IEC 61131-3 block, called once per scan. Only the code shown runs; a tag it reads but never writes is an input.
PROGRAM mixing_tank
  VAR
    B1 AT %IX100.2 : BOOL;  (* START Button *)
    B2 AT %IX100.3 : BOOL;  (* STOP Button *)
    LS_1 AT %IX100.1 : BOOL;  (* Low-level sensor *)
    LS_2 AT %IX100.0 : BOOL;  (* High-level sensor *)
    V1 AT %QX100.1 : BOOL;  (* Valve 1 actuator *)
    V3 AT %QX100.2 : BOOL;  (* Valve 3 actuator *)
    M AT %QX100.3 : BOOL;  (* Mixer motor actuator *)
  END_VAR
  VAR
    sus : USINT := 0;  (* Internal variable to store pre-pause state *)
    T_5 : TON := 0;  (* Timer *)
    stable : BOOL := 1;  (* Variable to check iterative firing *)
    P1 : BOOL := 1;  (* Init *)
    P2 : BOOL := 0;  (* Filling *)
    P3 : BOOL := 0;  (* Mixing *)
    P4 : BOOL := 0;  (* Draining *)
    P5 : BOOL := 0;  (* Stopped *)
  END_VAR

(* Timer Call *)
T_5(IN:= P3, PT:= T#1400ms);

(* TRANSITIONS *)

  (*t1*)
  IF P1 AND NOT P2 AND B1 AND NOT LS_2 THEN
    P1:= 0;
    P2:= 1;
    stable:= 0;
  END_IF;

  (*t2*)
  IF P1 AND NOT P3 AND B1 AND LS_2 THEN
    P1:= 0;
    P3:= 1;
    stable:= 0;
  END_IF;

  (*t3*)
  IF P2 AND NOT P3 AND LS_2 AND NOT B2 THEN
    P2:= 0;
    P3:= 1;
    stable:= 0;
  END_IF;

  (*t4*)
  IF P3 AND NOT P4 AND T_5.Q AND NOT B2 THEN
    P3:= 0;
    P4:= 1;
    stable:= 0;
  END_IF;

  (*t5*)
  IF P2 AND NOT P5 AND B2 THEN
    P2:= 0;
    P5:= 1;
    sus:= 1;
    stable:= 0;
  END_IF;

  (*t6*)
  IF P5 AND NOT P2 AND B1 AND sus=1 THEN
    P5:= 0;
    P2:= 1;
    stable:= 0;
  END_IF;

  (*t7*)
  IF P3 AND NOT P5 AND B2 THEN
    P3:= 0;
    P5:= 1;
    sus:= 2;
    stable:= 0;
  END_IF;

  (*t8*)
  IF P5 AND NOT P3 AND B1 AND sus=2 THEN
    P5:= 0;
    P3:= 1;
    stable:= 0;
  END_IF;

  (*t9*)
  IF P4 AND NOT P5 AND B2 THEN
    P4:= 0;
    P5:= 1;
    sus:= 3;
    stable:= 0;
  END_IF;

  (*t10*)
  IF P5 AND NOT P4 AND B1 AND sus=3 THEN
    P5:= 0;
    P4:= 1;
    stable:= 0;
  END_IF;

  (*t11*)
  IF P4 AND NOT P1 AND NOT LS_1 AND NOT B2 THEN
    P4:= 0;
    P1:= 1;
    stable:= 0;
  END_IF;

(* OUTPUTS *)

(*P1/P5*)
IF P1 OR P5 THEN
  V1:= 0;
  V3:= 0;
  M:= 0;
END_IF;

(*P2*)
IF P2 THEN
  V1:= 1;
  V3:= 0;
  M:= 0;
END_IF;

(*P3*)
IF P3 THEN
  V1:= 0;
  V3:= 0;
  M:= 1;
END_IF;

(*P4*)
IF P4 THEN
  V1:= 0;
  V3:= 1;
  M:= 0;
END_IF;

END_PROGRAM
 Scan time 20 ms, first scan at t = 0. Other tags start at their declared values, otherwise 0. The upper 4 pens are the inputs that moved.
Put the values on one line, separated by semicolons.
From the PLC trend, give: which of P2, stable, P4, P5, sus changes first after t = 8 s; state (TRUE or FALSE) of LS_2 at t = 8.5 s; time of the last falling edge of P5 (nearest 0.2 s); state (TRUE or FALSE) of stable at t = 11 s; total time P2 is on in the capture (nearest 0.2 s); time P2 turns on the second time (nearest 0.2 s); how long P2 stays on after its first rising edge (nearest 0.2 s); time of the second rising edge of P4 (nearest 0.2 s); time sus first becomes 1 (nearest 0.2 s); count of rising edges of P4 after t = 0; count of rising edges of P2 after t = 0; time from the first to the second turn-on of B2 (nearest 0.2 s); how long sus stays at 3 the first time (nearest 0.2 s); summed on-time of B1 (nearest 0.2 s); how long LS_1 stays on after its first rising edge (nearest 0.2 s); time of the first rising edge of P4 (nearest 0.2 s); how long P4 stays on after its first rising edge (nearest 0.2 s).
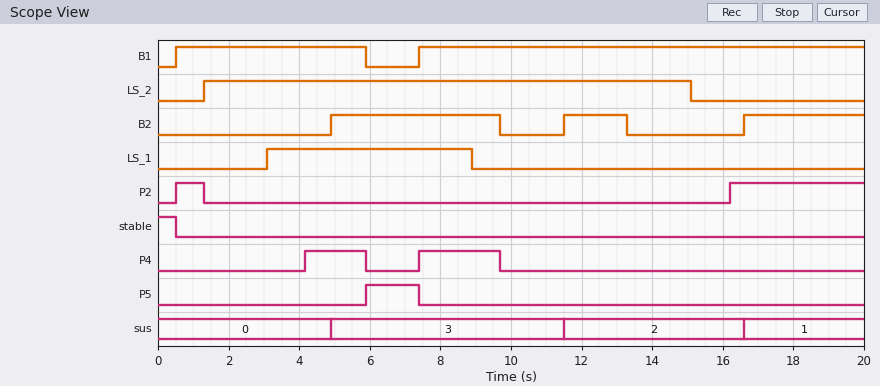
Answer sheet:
P4; TRUE; 7.4 s; FALSE; 4.6 s; 16.2 s; 0.8 s; 7.4 s; 16.6 s; 2; 2; 6.6 s; 6.6 s; 18.0 s; 5.8 s; 4.2 s; 1.8 s
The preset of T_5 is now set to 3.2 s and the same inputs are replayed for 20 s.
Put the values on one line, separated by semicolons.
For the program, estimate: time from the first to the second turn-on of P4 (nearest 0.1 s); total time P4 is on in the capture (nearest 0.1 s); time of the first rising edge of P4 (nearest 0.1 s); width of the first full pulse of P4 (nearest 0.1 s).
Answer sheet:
2.9 s; 3.7 s; 4.5 s; 1.4 s
